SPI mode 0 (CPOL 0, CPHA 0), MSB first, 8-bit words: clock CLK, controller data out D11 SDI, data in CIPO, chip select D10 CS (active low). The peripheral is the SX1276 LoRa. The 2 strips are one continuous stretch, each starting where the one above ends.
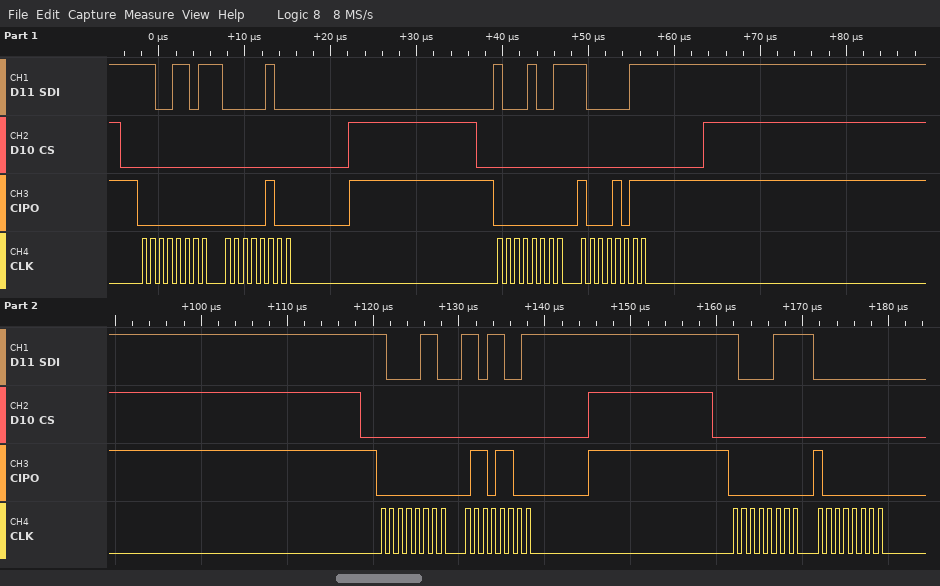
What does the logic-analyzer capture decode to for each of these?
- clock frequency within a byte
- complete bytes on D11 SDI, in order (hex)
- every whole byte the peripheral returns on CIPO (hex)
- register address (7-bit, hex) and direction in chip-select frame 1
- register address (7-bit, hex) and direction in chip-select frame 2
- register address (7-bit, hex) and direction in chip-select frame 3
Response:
1 MHz
0xCD 0x04 0x89 0x83 0x86 0xD9 0x87 0x00
0x00 0x04 0x00 0x8B 0x00 0x6C 0x00 0x80
0x4D write
0x09 write
0x06 write
